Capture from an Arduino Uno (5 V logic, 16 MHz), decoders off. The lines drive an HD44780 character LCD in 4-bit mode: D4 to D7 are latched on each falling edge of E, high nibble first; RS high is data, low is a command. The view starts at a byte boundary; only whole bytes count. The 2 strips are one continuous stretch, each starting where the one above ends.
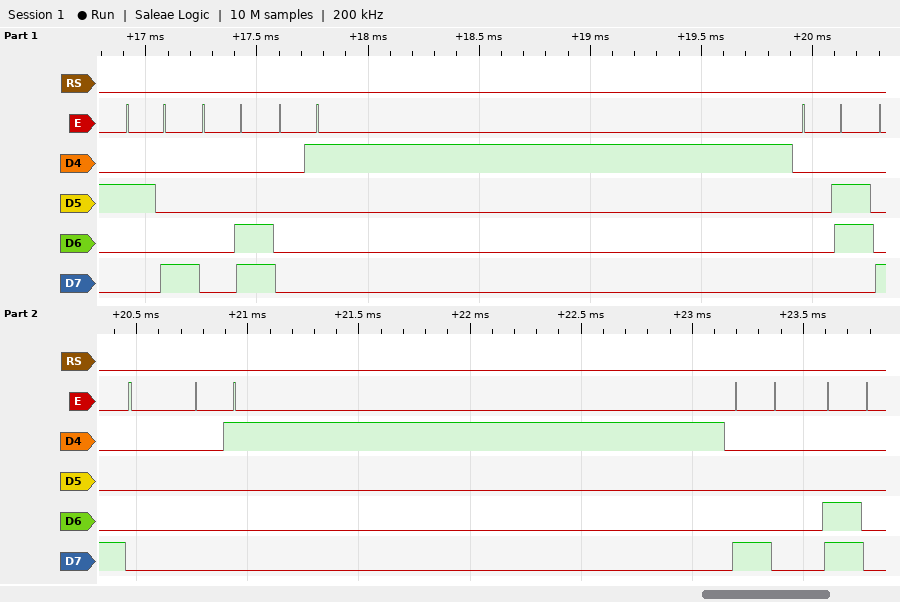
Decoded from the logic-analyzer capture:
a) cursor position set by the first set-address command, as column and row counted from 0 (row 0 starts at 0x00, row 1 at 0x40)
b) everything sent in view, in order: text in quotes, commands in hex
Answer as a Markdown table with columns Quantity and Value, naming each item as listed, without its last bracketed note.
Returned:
| Quantity | Value |
|---|---|
| cursor position set by the first set-address command, as column and row counted from 0 | column 0, row 0 |
| everything sent in view, in order: text in quotes, commands in hex | 0x28 0x0C 0x01 0x06 0x80 0x01 0x80 0xC0 |
